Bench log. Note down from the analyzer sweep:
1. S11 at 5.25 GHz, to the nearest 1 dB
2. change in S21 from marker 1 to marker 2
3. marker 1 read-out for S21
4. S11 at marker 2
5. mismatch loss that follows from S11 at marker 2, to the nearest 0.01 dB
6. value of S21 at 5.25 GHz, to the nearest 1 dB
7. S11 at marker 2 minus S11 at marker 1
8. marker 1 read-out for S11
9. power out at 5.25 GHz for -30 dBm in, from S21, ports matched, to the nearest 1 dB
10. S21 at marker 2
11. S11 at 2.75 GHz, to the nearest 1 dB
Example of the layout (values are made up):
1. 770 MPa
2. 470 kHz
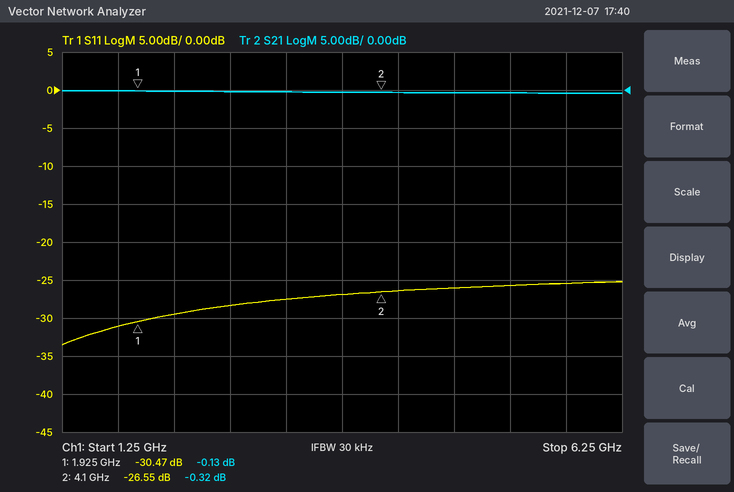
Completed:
1. -26 dB
2. -0.19 dB
3. -0.13 dB
4. -26.55 dB
5. 0.01 dB
6. 0 dB
7. 3.92 dB
8. -30.47 dB
9. -30 dBm
10. -0.32 dB
11. -28 dB
